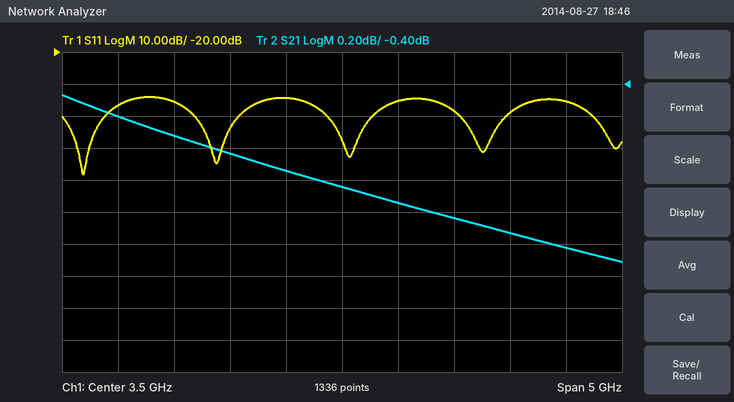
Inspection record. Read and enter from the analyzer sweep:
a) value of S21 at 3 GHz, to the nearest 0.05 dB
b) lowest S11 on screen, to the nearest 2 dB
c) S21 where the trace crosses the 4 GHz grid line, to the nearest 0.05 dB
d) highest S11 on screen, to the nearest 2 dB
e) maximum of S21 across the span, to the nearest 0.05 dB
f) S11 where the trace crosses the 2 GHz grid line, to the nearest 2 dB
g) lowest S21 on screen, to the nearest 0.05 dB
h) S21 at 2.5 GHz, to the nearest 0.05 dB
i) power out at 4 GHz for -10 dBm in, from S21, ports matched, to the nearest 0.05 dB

-0.95 dB
-58 dB
-1.15 dB
-34 dB
-0.45 dB
-36 dB
-1.50 dB
-0.85 dB
-11.15 dBm
